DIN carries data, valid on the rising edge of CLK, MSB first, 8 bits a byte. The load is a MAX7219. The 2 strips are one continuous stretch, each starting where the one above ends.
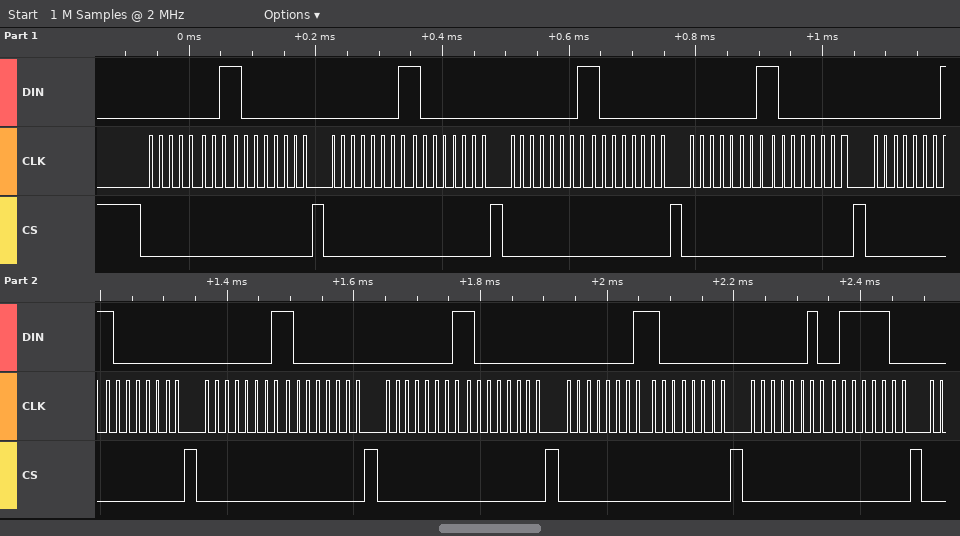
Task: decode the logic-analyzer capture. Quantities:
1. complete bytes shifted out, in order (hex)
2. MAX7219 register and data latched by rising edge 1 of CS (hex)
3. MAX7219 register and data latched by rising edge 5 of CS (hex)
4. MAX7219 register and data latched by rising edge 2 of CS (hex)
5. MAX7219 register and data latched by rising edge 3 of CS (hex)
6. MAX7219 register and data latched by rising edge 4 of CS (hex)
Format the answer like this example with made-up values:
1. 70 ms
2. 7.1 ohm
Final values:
1. 01 80 01 80 01 80 01 80 01 80 01 80 01 80 01 80 02 7C
2. register 0x1, data 0x80
3. register 0x1, data 0x80
4. register 0x1, data 0x80
5. register 0x1, data 0x80
6. register 0x1, data 0x80
